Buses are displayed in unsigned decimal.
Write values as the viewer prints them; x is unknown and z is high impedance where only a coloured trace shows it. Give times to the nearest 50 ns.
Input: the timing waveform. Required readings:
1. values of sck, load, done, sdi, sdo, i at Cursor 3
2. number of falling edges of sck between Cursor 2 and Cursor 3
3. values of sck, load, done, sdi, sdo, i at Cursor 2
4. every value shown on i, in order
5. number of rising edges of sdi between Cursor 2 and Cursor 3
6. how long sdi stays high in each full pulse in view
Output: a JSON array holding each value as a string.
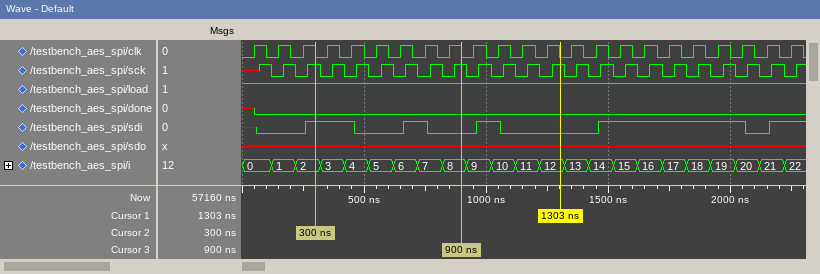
["sck=1, load=1, done=0, sdi=0, sdo=x, i=8", "6", "sck=1, load=1, done=0, sdi=1, sdo=x, i=2", "0, 1, 2, 3, 4, 5, 6, 7, 8, 9, 10, 11, 12, 13, 14, 15, 16, 17, 18, 19, 20, 21, 22", "1", "200 ns, 100 ns, 100 ns, 600 ns"]
